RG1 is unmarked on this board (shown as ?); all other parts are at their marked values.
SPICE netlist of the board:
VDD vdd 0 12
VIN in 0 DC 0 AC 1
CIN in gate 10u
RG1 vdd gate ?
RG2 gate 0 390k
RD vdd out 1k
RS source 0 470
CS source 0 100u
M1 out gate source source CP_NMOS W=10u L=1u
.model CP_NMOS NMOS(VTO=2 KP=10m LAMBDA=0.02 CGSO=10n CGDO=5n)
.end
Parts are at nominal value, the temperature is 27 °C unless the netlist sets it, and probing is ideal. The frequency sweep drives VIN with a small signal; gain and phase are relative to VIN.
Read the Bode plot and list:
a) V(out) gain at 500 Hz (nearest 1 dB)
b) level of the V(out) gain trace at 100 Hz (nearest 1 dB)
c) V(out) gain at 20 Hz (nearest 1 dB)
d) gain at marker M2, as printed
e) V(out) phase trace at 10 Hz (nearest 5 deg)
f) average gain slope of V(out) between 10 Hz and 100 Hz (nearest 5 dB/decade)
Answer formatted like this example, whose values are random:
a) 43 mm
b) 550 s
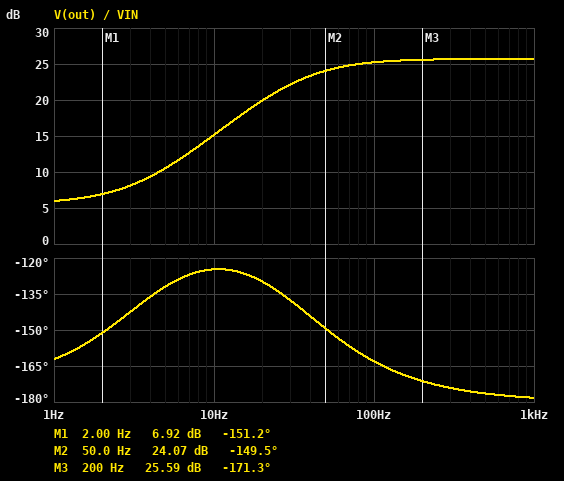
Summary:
a) 26 dB
b) 25 dB
c) 20 dB
d) 24.07 dB
e) -125 deg
f) 10 dB/decade
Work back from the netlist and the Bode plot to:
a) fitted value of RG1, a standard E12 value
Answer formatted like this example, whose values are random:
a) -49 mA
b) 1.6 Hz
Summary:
a) 1.2 MΩ
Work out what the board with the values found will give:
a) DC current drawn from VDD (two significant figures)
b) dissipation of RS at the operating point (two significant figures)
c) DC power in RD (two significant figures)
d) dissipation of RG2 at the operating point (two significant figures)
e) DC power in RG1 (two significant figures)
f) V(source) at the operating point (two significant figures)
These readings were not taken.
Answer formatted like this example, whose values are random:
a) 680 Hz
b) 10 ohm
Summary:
a) 1.7 mA
b) 1.3 mW
c) 2.7 mW
d) 22 µW
e) 68 µW
f) 780 mV
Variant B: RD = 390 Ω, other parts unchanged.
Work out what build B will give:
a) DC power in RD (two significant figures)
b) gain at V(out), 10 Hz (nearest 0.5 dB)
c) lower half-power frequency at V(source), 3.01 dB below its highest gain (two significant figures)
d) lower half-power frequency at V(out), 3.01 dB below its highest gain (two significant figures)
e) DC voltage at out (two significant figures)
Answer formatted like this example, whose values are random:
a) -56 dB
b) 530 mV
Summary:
a) 1.1 mW
b) 7.0 dB
c) 54 mHz
d) 35 Hz
e) 11 V
